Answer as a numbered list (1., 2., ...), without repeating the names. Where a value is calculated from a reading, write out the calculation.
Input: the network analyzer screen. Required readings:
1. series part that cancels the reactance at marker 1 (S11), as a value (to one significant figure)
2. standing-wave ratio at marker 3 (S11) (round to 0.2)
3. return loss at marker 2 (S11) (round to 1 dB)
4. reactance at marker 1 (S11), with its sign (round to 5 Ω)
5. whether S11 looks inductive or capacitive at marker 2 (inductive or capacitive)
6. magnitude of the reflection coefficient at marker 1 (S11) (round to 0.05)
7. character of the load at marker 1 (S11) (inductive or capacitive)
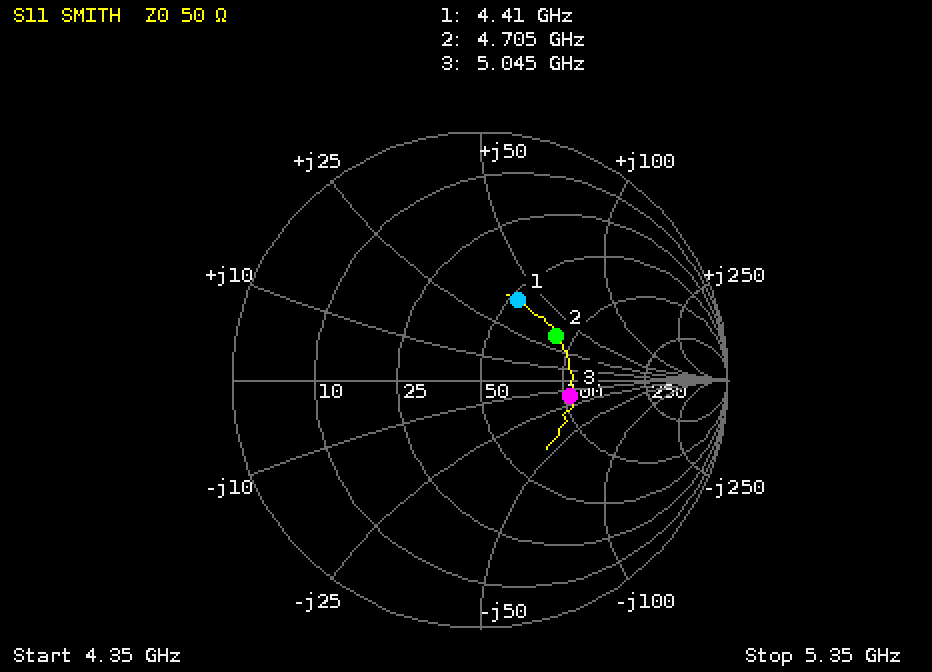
1. C = 1/(2π × 4.41 GHz × 40 Ω) ≈ 902 fF, so 900 fF to one significant figure
2. 2.2
3. 9 dB
4. +40 Ω
5. inductive
6. 0.35
7. inductive
